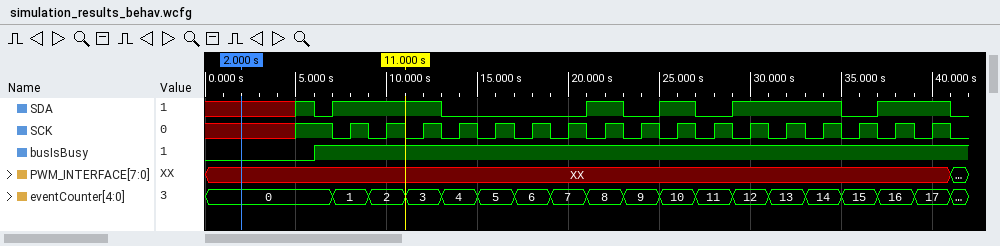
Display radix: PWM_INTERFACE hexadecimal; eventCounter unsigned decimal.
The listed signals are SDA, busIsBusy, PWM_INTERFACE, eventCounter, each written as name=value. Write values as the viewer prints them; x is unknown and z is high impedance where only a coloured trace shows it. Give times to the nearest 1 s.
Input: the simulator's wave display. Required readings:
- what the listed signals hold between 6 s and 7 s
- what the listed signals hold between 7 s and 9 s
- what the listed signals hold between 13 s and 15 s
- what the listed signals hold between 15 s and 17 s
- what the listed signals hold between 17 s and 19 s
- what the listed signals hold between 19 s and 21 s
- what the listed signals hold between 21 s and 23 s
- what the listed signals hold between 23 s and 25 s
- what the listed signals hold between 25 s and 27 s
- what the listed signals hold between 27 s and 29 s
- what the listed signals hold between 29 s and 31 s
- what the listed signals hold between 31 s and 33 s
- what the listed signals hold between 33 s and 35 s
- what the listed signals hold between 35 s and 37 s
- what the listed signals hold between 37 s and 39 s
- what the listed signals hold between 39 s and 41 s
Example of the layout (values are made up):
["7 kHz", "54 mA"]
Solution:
["SDA=0, busIsBusy=1, PWM_INTERFACE=XX, eventCounter=0", "SDA=1, busIsBusy=1, PWM_INTERFACE=XX, eventCounter=1", "SDA=0, busIsBusy=1, PWM_INTERFACE=XX, eventCounter=4", "SDA=0, busIsBusy=1, PWM_INTERFACE=XX, eventCounter=5", "SDA=0, busIsBusy=1, PWM_INTERFACE=XX, eventCounter=6", "SDA=0, busIsBusy=1, PWM_INTERFACE=XX, eventCounter=7", "SDA=1, busIsBusy=1, PWM_INTERFACE=XX, eventCounter=8", "SDA=0, busIsBusy=1, PWM_INTERFACE=XX, eventCounter=9", "SDA=1, busIsBusy=1, PWM_INTERFACE=XX, eventCounter=10", "SDA=0, busIsBusy=1, PWM_INTERFACE=XX, eventCounter=11", "SDA=1, busIsBusy=1, PWM_INTERFACE=XX, eventCounter=12", "SDA=1, busIsBusy=1, PWM_INTERFACE=XX, eventCounter=13", "SDA=1, busIsBusy=1, PWM_INTERFACE=XX, eventCounter=14", "SDA=0, busIsBusy=1, PWM_INTERFACE=XX, eventCounter=15", "SDA=1, busIsBusy=1, PWM_INTERFACE=XX, eventCounter=16", "SDA=1, busIsBusy=1, PWM_INTERFACE=XX, eventCounter=17"]
